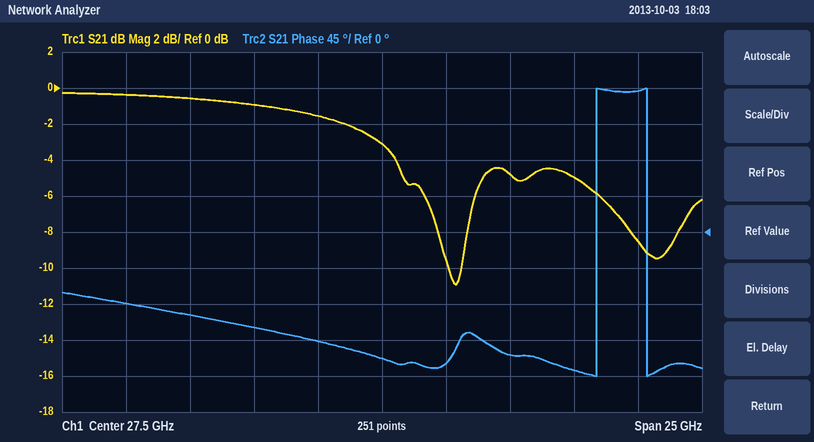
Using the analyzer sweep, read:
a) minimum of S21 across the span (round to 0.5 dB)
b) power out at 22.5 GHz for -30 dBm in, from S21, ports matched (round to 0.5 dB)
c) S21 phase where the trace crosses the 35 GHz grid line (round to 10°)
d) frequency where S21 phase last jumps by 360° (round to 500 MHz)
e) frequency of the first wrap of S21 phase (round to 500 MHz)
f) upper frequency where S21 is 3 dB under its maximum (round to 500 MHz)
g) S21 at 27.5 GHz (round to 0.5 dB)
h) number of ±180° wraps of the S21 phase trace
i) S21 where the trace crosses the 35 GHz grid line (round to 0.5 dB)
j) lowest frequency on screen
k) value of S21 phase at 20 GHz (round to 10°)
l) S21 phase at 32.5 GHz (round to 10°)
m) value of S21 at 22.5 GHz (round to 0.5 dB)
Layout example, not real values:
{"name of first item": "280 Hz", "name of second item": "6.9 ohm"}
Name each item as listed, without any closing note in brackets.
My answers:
{"minimum of S21 across the span": "-11.0 dB", "power out at 22.5 GHz for -30 dBm in, from S21, ports matched": "-31.0 dBm", "S21 phase where the trace crosses the 35 GHz grid line": "-170°", "frequency where S21 phase last jumps by 360°": "38.0 GHz", "frequency of the first wrap of S21 phase": "36.0 GHz", "upper frequency where S21 is 3 dB under its maximum": "27.5 GHz", "S21 at 27.5 GHz": "-3.0 dB", "number of ±180° wraps of the S21 phase trace": "2", "S21 where the trace crosses the 35 GHz grid line": "-5.0 dB", "lowest frequency on screen": "15 GHz", "value of S21 phase at 20 GHz": "-100°", "S21 phase at 32.5 GHz": "-150°", "value of S21 at 22.5 GHz": "-1.0 dB"}
